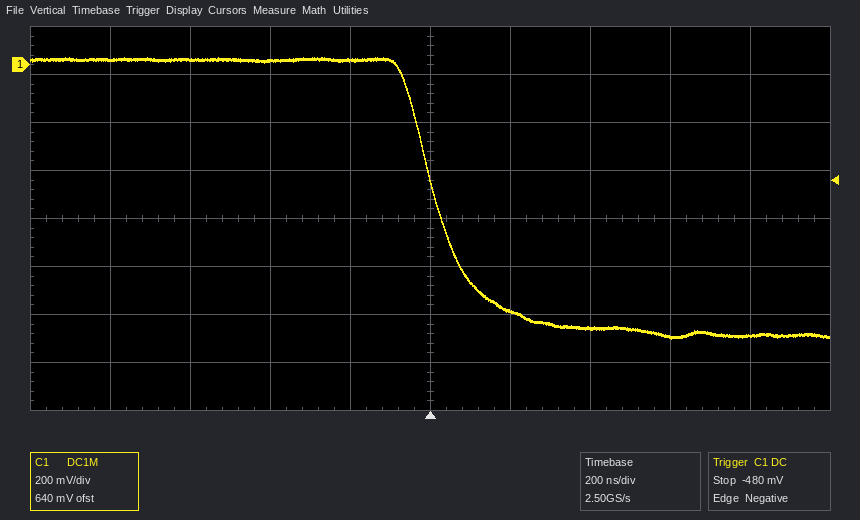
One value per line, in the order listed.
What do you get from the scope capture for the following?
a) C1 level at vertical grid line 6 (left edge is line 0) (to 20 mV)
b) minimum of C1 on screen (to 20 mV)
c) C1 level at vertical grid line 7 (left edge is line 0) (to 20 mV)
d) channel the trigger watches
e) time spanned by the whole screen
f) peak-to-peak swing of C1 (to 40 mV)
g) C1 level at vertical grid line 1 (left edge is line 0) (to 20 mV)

-1.02 V
-1.14 V
-1.10 V
C1
2 µs
1.16 V
20 mV
